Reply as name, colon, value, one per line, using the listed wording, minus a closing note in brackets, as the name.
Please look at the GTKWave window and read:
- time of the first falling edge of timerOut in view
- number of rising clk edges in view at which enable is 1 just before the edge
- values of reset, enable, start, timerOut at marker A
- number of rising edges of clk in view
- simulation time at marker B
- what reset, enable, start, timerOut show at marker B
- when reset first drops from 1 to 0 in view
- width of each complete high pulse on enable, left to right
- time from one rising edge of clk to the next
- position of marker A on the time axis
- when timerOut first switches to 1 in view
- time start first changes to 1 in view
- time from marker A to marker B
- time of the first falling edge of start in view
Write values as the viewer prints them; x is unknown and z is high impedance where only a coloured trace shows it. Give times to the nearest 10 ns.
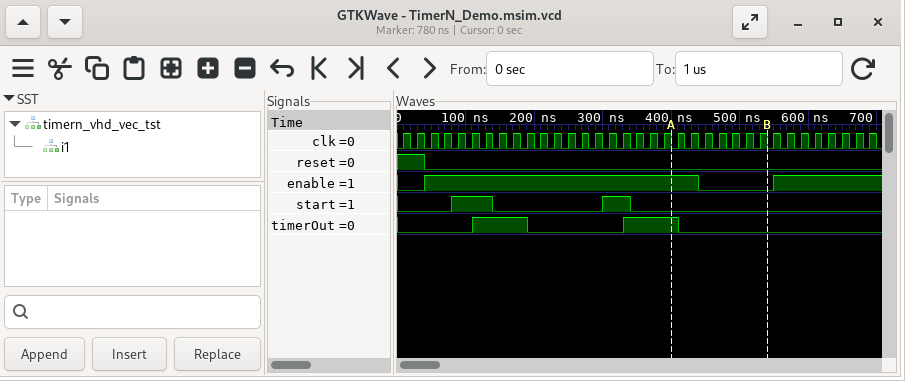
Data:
time of the first falling edge of timerOut in view: 190 ns
number of rising clk edges in view at which enable is 1 just before the edge: 27
values of reset, enable, start, timerOut at marker A: reset=0, enable=1, start=0, timerOut=1
number of rising edges of clk in view: 35
simulation time at marker B: 540 ns
what reset, enable, start, timerOut show at marker B: reset=0, enable=0, start=0, timerOut=0
when reset first drops from 1 to 0 in view: 40 ns
width of each complete high pulse on enable, left to right: 400 ns
time from one rising edge of clk to the next: 20 ns
position of marker A on the time axis: 400 ns
when timerOut first switches to 1 in view: 110 ns
time start first changes to 1 in view: 80 ns
time from marker A to marker B: 140 ns
time of the first falling edge of start in view: 140 ns
